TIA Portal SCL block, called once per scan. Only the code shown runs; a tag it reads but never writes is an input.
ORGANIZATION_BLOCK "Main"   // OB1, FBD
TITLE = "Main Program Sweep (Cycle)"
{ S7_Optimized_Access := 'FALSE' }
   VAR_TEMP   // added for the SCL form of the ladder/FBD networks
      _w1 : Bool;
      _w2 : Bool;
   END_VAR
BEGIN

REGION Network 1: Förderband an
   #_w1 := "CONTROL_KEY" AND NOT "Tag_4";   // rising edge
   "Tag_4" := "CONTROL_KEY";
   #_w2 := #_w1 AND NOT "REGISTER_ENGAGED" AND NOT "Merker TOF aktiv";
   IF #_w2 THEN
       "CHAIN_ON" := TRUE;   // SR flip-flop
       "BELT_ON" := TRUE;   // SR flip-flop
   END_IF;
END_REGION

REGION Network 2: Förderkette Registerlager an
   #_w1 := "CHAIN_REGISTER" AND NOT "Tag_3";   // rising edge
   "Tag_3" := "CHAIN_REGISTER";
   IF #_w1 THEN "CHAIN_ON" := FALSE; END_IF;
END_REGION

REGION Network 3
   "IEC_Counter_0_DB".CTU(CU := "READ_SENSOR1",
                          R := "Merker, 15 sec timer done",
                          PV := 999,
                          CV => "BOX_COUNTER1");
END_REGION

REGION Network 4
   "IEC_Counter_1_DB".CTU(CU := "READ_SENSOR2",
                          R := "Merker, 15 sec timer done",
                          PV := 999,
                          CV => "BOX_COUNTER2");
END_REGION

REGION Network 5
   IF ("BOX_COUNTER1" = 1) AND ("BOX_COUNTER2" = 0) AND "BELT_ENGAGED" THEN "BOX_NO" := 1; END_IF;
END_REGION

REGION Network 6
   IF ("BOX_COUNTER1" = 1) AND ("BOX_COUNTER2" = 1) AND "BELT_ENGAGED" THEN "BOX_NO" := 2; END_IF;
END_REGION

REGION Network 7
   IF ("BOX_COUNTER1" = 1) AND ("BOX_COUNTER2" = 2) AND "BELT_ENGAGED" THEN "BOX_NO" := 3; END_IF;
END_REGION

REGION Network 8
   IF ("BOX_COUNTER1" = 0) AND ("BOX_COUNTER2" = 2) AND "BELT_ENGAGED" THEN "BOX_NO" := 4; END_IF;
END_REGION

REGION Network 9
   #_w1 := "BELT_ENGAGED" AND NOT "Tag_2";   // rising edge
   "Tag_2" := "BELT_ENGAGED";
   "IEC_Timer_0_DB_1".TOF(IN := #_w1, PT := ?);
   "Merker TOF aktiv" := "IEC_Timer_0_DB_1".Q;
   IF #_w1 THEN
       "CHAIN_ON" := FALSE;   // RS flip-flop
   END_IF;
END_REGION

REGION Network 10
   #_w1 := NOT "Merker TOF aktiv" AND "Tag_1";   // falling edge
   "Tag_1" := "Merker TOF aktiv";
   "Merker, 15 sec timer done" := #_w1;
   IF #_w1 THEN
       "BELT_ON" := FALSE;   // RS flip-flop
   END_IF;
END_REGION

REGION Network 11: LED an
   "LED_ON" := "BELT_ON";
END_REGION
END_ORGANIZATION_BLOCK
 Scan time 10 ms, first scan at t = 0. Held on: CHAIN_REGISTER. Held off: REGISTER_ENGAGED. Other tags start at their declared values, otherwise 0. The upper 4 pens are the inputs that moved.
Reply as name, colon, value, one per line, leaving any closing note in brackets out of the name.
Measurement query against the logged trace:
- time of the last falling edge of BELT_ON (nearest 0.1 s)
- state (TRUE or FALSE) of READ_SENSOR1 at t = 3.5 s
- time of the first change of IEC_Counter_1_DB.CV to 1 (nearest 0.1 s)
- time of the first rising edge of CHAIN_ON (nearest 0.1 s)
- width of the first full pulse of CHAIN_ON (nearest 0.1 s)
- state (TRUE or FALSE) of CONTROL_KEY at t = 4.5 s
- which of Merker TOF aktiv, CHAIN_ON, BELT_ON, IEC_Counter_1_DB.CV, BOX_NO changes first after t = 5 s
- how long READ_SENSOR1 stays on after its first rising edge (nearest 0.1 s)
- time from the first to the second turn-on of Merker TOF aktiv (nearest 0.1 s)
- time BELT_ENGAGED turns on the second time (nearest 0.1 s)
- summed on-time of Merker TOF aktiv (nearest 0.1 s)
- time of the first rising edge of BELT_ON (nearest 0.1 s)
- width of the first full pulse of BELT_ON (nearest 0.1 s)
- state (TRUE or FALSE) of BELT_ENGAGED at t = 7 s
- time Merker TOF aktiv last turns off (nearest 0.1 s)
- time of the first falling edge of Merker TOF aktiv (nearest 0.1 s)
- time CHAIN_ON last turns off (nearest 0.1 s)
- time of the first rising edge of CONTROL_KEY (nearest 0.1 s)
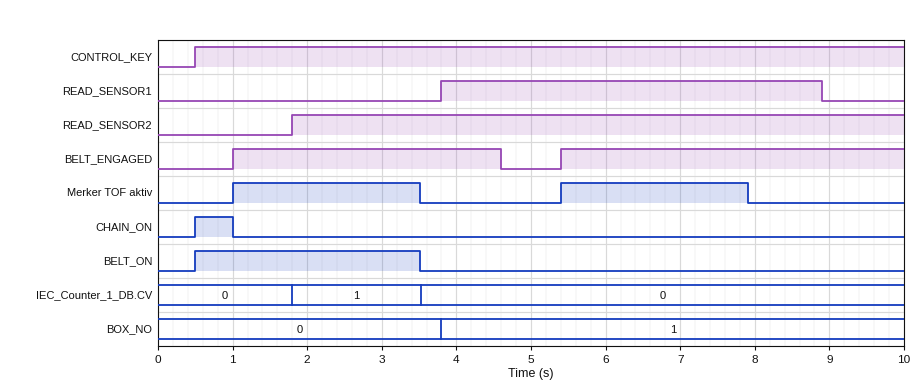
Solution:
time of the last falling edge of BELT_ON: 3.5 s
state (TRUE or FALSE) of READ_SENSOR1 at t = 3.5 s: FALSE
time of the first change of IEC_Counter_1_DB.CV to 1: 1.8 s
time of the first rising edge of CHAIN_ON: 0.5 s
width of the first full pulse of CHAIN_ON: 0.5 s
state (TRUE or FALSE) of CONTROL_KEY at t = 4.5 s: TRUE
which of Merker TOF aktiv, CHAIN_ON, BELT_ON, IEC_Counter_1_DB.CV, BOX_NO changes first after t = 5 s: Merker TOF aktiv
how long READ_SENSOR1 stays on after its first rising edge: 5.1 s
time from the first to the second turn-on of Merker TOF aktiv: 4.4 s
time BELT_ENGAGED turns on the second time: 5.4 s
summed on-time of Merker TOF aktiv: 5.0 s
time of the first rising edge of BELT_ON: 0.5 s
width of the first full pulse of BELT_ON: 3.0 s
state (TRUE or FALSE) of BELT_ENGAGED at t = 7 s: TRUE
time Merker TOF aktiv last turns off: 7.9 s
time of the first falling edge of Merker TOF aktiv: 3.5 s
time CHAIN_ON last turns off: 1.0 s
time of the first rising edge of CONTROL_KEY: 0.5 s
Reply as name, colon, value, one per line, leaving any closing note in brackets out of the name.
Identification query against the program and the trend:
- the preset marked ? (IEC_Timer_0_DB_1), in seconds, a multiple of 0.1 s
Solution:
the preset marked ? (IEC_Timer_0_DB_1), in seconds, a multiple of 0.1 s: 2.5 s
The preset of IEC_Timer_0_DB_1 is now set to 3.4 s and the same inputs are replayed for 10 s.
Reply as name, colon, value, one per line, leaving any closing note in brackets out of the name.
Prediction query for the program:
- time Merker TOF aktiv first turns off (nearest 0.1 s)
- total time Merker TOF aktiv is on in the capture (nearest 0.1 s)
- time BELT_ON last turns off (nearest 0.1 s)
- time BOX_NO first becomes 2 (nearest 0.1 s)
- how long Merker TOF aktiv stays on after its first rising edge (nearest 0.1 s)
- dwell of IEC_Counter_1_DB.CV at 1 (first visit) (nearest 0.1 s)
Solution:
time Merker TOF aktiv first turns off: 4.4 s
total time Merker TOF aktiv is on in the capture: 6.8 s
time BELT_ON last turns off: 4.4 s
time BOX_NO first becomes 2: 3.8 s
how long Merker TOF aktiv stays on after its first rising edge: 3.4 s
dwell of IEC_Counter_1_DB.CV at 1 (first visit): 2.6 s
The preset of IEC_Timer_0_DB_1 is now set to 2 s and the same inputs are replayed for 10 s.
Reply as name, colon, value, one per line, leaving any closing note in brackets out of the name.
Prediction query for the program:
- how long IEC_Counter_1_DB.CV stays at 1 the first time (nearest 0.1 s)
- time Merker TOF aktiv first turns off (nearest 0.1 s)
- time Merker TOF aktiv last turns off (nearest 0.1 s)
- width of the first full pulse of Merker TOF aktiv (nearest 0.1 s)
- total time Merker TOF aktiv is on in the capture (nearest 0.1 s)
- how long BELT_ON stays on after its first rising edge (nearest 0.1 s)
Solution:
how long IEC_Counter_1_DB.CV stays at 1 the first time: 1.2 s
time Merker TOF aktiv first turns off: 3.0 s
time Merker TOF aktiv last turns off: 7.4 s
width of the first full pulse of Merker TOF aktiv: 2.0 s
total time Merker TOF aktiv is on in the capture: 4.0 s
how long BELT_ON stays on after its first rising edge: 2.5 s
